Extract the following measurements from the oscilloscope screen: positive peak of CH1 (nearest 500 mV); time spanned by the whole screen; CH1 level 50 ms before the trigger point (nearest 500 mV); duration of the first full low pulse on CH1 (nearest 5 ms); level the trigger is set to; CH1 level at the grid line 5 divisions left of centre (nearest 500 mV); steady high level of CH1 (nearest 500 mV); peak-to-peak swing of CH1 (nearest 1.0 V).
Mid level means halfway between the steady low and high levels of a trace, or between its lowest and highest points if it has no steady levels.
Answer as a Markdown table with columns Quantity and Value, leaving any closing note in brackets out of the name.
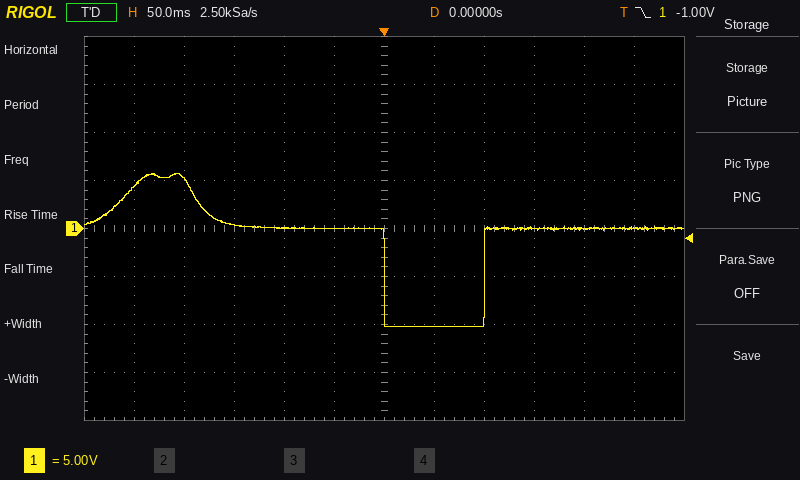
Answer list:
| Quantity | Value |
|---|---|
| positive peak of CH1 | 5.5 V |
| time spanned by the whole screen | 600 ms |
| CH1 level 50 ms before the trigger point | 0.0 V |
| duration of the first full low pulse on CH1 | 100 ms |
| level the trigger is set to | -1.00 V |
| CH1 level at the grid line 5 divisions left of centre | 4.5 V |
| steady high level of CH1 | 0.0 V |
| peak-to-peak swing of CH1 | 16.0 V |
